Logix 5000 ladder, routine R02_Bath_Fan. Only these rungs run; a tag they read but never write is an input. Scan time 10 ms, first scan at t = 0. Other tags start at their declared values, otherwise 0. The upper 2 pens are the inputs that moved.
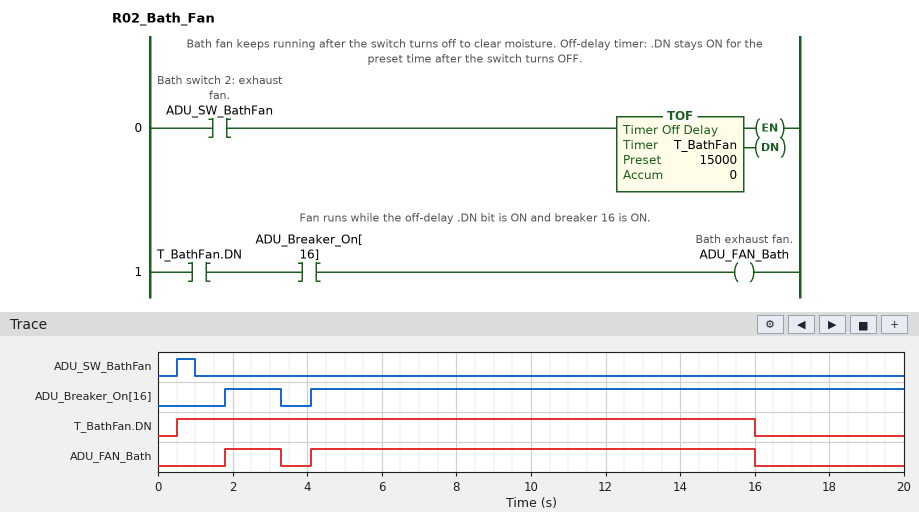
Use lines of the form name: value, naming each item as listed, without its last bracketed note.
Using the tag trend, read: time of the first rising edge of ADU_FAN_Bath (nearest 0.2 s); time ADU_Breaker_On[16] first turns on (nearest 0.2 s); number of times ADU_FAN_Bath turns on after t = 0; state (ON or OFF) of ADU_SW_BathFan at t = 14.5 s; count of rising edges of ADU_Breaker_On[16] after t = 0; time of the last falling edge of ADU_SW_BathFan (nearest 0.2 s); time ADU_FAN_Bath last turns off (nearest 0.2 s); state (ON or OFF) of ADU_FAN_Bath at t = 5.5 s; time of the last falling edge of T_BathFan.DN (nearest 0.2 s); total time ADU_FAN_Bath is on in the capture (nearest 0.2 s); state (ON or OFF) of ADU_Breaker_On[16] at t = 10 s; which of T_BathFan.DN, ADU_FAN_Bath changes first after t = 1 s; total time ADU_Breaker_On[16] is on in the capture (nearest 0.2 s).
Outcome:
time of the first rising edge of ADU_FAN_Bath: 1.8 s
time ADU_Breaker_On[16] first turns on: 1.8 s
number of times ADU_FAN_Bath turns on after t = 0: 2
state (ON or OFF) of ADU_SW_BathFan at t = 14.5 s: OFF
count of rising edges of ADU_Breaker_On[16] after t = 0: 2
time of the last falling edge of ADU_SW_BathFan: 1.0 s
time ADU_FAN_Bath last turns off: 16.0 s
state (ON or OFF) of ADU_FAN_Bath at t = 5.5 s: ON
time of the last falling edge of T_BathFan.DN: 16.0 s
total time ADU_FAN_Bath is on in the capture: 13.4 s
state (ON or OFF) of ADU_Breaker_On[16] at t = 10 s: ON
which of T_BathFan.DN, ADU_FAN_Bath changes first after t = 1 s: ADU_FAN_Bath
total time ADU_Breaker_On[16] is on in the capture: 17.4 s
